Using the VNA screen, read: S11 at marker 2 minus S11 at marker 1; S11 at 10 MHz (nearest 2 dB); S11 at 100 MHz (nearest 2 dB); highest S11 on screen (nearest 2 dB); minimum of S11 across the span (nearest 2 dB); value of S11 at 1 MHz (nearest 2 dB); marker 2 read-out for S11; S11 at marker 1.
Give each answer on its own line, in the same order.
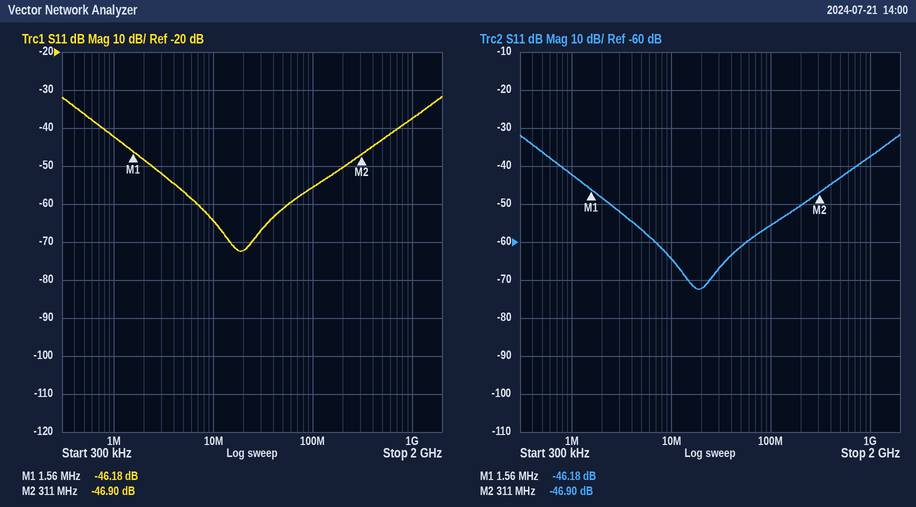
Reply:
-0.72 dB
-64 dB
-56 dB
-32 dB
-72 dB
-42 dB
-46.90 dB
-46.18 dB
